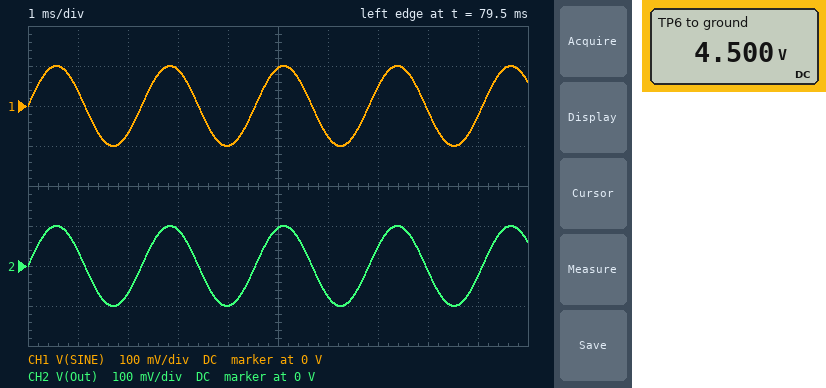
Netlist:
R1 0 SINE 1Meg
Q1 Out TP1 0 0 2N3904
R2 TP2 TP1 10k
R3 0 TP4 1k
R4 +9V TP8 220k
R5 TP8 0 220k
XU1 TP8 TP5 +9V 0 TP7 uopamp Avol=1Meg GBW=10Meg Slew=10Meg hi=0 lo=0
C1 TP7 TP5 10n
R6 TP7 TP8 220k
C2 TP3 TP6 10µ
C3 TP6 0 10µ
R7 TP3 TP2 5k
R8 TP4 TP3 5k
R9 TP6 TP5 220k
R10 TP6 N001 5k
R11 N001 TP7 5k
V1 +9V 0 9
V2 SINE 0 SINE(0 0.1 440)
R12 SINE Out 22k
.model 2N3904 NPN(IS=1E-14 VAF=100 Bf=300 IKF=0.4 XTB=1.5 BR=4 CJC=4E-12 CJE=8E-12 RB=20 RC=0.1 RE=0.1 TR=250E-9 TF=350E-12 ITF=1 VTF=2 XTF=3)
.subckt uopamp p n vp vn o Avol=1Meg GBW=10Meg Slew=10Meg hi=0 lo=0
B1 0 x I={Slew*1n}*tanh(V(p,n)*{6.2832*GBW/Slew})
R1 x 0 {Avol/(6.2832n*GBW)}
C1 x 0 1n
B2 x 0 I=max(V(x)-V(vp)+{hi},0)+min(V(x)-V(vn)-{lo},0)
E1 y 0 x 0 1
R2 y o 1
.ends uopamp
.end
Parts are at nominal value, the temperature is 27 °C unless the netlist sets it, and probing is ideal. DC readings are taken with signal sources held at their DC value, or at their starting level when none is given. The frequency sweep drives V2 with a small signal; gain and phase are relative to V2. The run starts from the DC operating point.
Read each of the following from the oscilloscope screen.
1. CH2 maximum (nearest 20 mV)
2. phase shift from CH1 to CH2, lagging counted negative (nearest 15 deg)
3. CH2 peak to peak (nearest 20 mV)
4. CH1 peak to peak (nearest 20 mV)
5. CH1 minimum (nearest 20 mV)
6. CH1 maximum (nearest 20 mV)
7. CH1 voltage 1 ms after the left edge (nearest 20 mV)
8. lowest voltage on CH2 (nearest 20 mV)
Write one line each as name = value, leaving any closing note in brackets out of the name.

CH2 maximum = 100 mV
phase shift from CH1 to CH2, lagging counted negative = 0 deg
CH2 peak to peak = 200 mV
CH1 peak to peak = 200 mV
CH1 minimum = -100 mV
CH1 maximum = 100 mV
CH1 voltage 1 ms after the left edge = 40 mV
lowest voltage on CH2 = -100 mV
